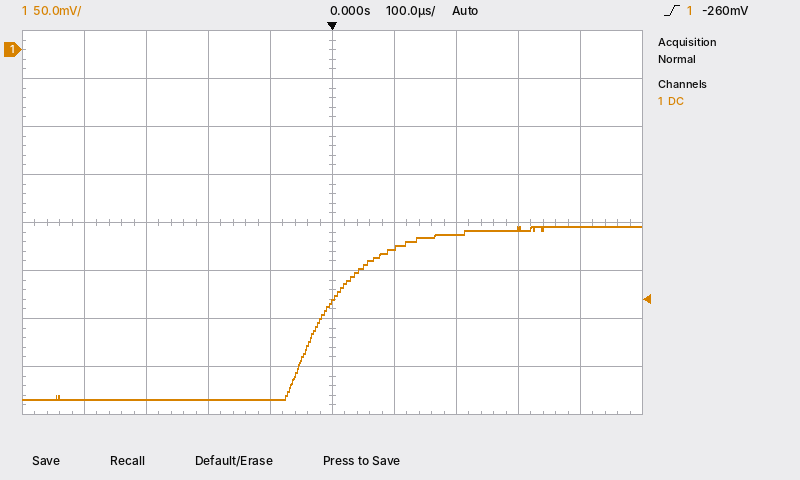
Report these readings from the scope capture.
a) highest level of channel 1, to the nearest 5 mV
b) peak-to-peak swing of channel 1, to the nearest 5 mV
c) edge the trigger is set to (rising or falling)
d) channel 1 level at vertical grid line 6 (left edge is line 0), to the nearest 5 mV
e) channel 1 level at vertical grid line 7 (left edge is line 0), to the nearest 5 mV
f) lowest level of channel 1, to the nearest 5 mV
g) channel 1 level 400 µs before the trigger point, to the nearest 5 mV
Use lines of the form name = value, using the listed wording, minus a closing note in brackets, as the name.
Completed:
highest level of channel 1, to the nearest 5 mV = -185 mV
peak-to-peak swing of channel 1, to the nearest 5 mV = 180 mV
edge the trigger is set to = rising
channel 1 level at vertical grid line 6 (left edge is line 0), to the nearest 5 mV = -205 mV
channel 1 level at vertical grid line 7 (left edge is line 0), to the nearest 5 mV = -190 mV
lowest level of channel 1, to the nearest 5 mV = -365 mV
channel 1 level 400 µs before the trigger point, to the nearest 5 mV = -365 mV
